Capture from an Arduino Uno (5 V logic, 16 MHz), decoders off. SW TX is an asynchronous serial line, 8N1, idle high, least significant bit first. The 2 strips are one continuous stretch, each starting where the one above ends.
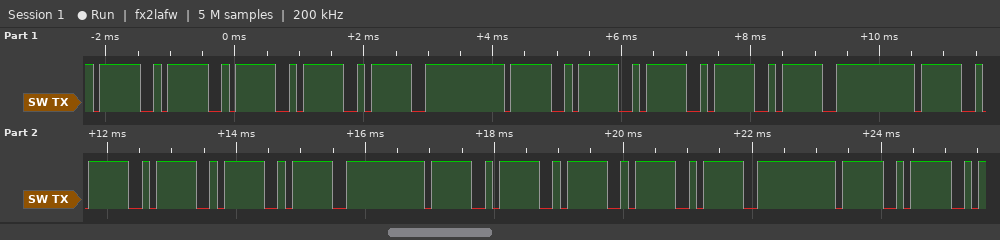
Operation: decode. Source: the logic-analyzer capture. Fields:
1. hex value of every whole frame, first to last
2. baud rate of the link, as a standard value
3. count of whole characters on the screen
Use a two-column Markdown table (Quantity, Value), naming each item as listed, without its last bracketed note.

| Quantity | Value |
|---|---|
| hex value of every whole frame, first to last | 3F 3F 3F 3F 3F 3F 3F 3F 3F 3F 3F 3F 3F 3F 3F 3F 3F 3F 3F 3F 3F 3F |
| baud rate of the link, as a standard value | 9600 baud |
| count of whole characters on the screen | 22 |
